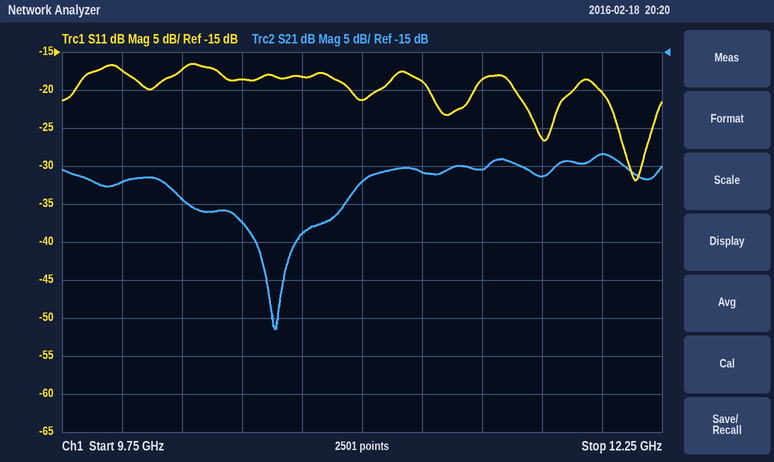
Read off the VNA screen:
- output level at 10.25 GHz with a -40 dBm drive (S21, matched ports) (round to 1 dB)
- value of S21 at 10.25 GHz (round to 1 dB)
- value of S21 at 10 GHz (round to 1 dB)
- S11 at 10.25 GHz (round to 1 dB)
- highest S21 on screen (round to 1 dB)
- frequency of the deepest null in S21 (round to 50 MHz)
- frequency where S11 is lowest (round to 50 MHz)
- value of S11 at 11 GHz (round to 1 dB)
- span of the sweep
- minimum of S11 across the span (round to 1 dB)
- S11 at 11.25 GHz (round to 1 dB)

-74 dBm
-34 dB
-32 dB
-17 dB
-28 dB
10.65 GHz
12.15 GHz
-21 dB
2.5 GHz
-32 dB
-19 dB
